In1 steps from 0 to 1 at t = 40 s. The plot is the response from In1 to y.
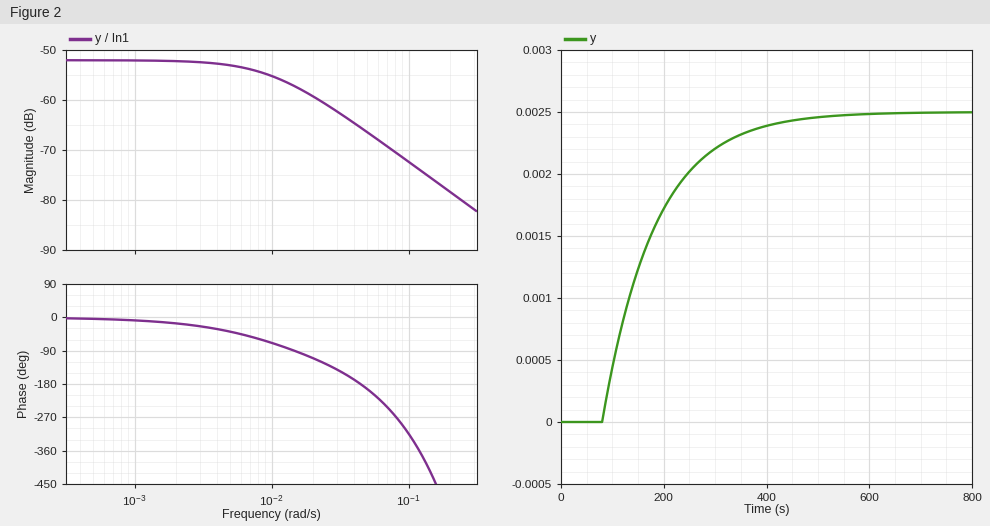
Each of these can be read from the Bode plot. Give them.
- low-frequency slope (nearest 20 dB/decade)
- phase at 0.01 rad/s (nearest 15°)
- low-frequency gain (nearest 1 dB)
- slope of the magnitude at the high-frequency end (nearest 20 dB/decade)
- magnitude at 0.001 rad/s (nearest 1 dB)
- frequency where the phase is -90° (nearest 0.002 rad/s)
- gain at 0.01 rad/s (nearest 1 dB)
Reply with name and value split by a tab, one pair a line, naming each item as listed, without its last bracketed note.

low-frequency slope	0 dB/decade
phase at 0.01 rad/s	-75°
low-frequency gain	-52 dB
slope of the magnitude at the high-frequency end	-20 dB/decade
magnitude at 0.001 rad/s	-52 dB
frequency where the phase is -90°	0.014 rad/s
gain at 0.01 rad/s	-55 dB
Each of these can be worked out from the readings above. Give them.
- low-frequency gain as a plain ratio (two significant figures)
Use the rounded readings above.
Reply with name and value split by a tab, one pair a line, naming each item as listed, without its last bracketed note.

low-frequency gain as a plain ratio	0.0025
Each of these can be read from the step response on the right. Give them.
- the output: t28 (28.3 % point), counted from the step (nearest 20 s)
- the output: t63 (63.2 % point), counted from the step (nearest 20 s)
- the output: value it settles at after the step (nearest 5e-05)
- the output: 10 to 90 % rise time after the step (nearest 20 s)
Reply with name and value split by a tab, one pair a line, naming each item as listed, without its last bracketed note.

the output: t28 (28.3 % point), counted from the step	80 s
the output: t63 (63.2 % point), counted from the step	140 s
the output: value it settles at after the step	0.00250
the output: 10 to 90 % rise time after the step	220 s
